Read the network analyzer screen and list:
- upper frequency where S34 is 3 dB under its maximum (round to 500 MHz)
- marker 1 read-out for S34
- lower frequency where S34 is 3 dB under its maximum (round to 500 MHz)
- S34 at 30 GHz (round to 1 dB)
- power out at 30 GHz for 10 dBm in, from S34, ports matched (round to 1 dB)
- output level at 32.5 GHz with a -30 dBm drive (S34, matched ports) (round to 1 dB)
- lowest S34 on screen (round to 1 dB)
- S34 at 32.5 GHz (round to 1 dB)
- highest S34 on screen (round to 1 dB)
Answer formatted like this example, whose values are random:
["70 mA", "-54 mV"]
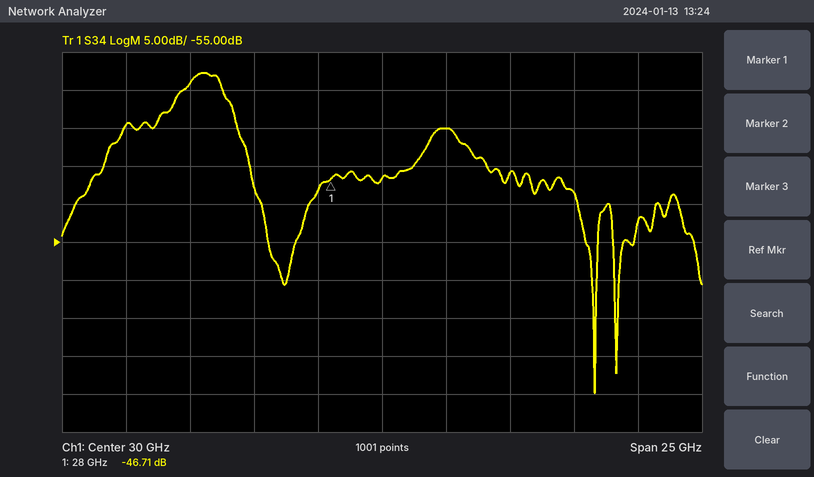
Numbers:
["24.0 GHz", "-46.71 dB", "22.0 GHz", "-47 dB", "-37 dBm", "-70 dBm", "-75 dB", "-40 dB", "-33 dB"]
